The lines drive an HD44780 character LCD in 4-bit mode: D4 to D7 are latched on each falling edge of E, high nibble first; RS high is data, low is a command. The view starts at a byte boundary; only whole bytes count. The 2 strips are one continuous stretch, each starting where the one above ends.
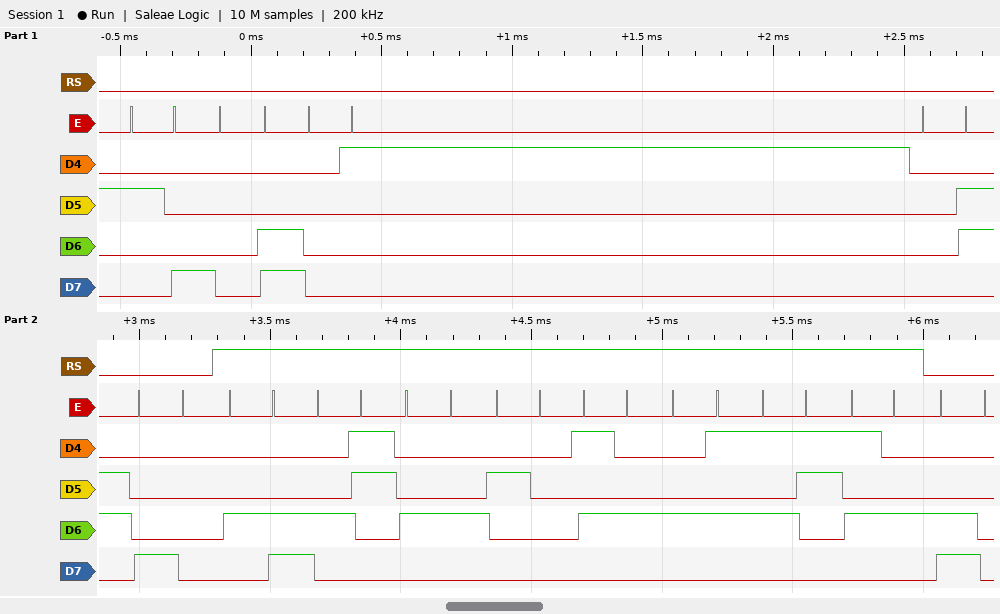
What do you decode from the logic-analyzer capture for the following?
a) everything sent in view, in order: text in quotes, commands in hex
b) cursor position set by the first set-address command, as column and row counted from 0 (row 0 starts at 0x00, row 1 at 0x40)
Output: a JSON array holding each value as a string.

["0x28 0x0C 0x01 0x06 0x80 \"LCD TEST\" 0xC0", "column 0, row 0"]
